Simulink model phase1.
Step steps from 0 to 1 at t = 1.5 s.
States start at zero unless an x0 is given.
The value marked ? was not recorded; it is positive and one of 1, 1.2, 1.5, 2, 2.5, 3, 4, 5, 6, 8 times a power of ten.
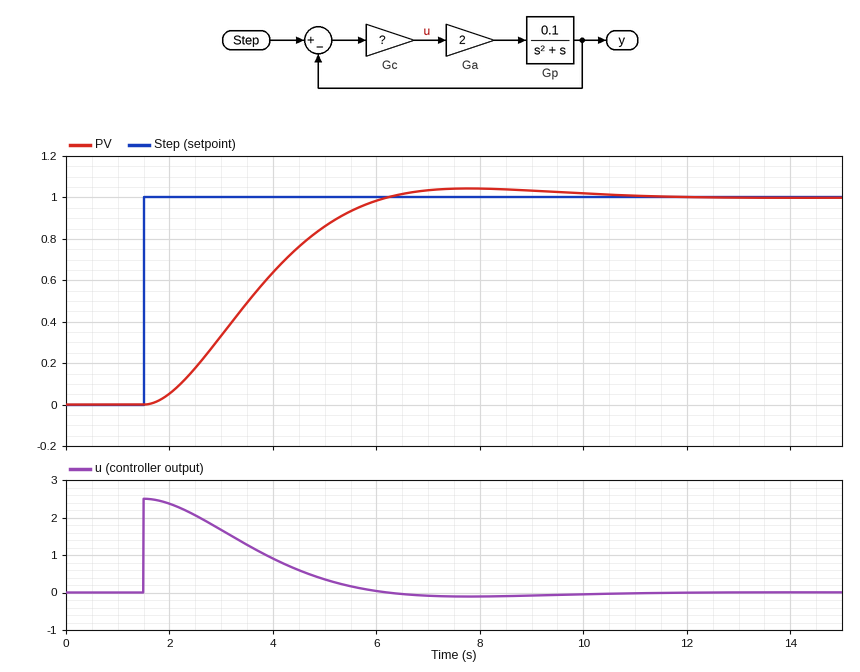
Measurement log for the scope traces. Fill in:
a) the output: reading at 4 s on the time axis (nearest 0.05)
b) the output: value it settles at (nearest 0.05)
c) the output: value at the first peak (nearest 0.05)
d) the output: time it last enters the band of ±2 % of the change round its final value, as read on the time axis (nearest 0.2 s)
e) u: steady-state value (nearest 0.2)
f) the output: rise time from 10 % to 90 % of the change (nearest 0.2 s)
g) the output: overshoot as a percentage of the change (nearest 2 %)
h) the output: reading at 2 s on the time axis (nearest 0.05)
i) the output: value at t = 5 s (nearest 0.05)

0.65
1.00
1.05
10.0 s
0.0
3.0 s
4 %
0.05
0.85
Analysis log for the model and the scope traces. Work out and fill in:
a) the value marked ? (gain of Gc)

2.5
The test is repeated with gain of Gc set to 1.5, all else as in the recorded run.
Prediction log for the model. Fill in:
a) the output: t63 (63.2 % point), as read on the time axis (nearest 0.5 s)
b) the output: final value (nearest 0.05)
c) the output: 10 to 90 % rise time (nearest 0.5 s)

5.0 s
1.00
5.5 s
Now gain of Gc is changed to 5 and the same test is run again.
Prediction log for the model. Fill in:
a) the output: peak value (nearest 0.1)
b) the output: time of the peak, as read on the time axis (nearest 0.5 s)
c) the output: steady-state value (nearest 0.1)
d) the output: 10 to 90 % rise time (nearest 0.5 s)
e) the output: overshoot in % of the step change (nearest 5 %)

1.2
5.0 s
1.0
1.5 s
15 %
